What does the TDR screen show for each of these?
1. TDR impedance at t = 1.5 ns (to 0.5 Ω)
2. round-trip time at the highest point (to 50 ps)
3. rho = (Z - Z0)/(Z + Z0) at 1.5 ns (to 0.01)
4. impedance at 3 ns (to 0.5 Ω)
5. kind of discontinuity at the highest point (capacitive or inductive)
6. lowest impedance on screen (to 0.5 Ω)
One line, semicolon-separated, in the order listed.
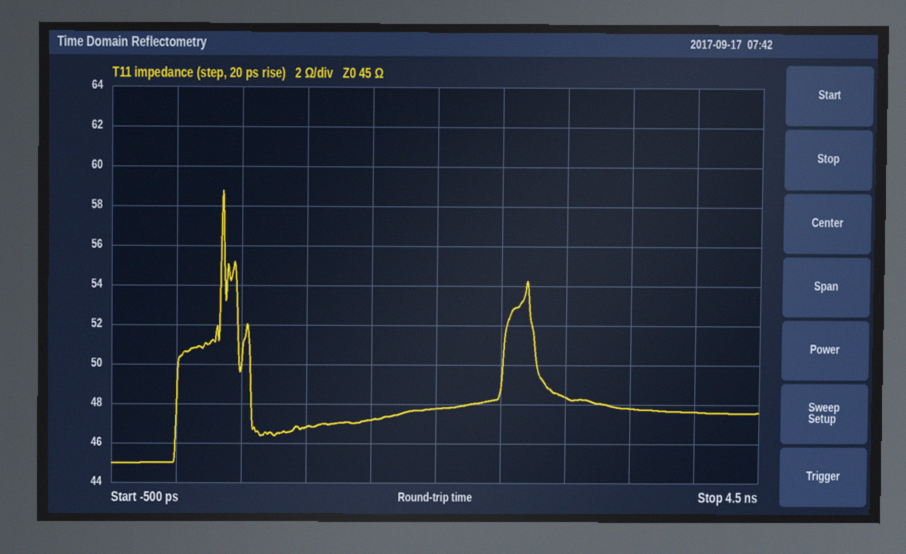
47.0 Ω; 350 ps; +0.02; 48.5 Ω; inductive; 45.0 Ω
